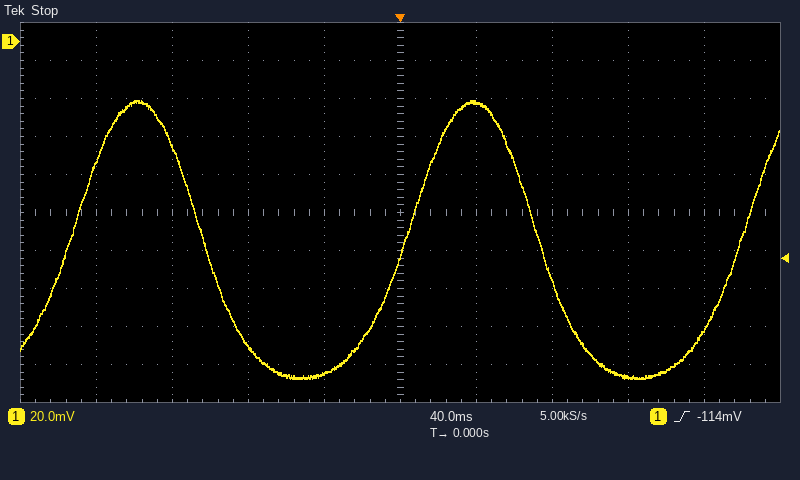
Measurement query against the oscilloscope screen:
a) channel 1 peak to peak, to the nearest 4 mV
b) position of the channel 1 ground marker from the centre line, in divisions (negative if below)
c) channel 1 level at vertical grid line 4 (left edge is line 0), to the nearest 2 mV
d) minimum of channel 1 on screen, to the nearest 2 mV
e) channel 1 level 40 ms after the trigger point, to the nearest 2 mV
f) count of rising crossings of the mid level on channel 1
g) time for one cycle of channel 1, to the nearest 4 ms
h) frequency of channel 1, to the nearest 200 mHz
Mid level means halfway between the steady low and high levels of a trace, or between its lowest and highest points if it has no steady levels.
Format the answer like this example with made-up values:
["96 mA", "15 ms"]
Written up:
["148 mV", "+4.5 div", "-174 mV", "-178 mV", "-32 mV", "3", "176 ms", "5.6 Hz"]
